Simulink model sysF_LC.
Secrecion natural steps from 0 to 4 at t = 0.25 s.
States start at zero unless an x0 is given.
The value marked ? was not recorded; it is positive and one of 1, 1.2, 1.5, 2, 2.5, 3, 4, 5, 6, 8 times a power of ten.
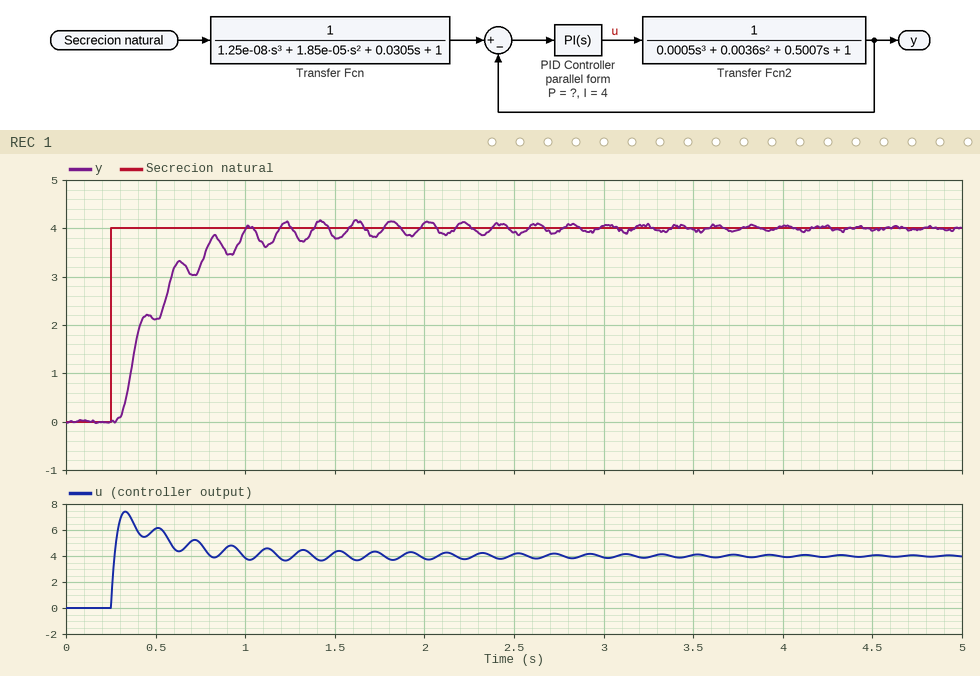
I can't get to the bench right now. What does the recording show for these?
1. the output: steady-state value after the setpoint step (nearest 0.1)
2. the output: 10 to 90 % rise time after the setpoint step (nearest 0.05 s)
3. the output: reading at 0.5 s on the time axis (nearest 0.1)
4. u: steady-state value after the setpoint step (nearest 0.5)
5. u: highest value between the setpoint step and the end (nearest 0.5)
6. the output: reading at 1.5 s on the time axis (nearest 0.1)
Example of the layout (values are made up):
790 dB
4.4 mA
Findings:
4.0
0.45 s
2.1
4.0
7.5
3.8
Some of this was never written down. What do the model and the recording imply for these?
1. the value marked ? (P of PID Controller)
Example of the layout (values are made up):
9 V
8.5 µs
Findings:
2
